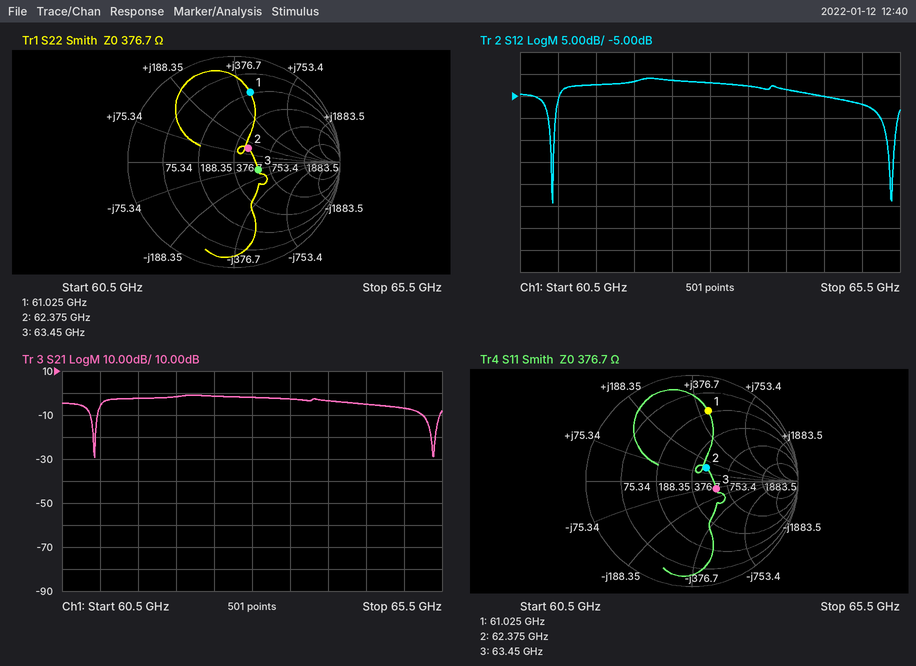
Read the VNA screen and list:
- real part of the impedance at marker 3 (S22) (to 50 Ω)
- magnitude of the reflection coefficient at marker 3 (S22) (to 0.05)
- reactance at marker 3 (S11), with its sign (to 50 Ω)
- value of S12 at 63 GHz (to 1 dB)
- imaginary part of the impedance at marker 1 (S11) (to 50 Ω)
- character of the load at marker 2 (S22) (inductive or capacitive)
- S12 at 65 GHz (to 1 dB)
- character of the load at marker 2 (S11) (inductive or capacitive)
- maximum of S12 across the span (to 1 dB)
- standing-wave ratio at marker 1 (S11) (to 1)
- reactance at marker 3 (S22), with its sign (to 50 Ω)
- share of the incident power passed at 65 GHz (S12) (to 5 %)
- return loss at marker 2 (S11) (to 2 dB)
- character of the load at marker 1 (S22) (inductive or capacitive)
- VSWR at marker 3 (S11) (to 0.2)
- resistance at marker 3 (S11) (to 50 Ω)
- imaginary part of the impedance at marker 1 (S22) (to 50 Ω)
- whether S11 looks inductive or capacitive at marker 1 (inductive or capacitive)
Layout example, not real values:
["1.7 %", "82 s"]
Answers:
["600 Ω", "0.25", "-100 Ω", "-2 dB", "+450 Ω", "inductive", "-7 dB", "inductive", "-1 dB", "5", "-100 Ω", "20 %", "14 dB", "inductive", "1.6", "600 Ω", "+450 Ω", "inductive"]
